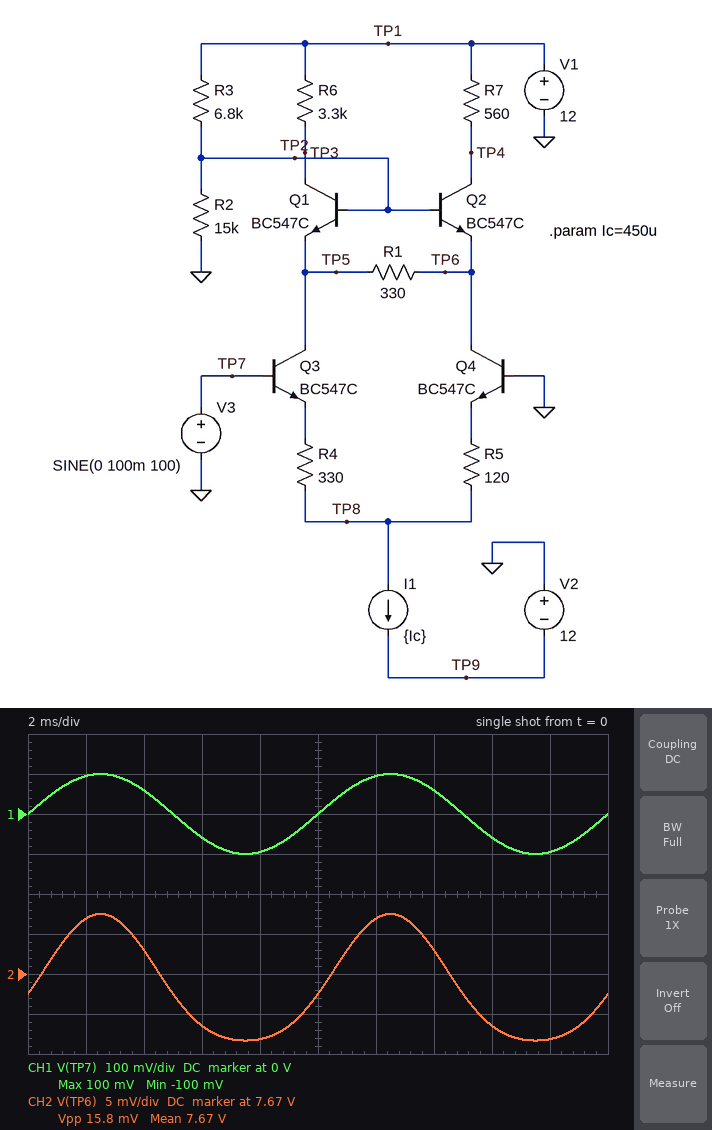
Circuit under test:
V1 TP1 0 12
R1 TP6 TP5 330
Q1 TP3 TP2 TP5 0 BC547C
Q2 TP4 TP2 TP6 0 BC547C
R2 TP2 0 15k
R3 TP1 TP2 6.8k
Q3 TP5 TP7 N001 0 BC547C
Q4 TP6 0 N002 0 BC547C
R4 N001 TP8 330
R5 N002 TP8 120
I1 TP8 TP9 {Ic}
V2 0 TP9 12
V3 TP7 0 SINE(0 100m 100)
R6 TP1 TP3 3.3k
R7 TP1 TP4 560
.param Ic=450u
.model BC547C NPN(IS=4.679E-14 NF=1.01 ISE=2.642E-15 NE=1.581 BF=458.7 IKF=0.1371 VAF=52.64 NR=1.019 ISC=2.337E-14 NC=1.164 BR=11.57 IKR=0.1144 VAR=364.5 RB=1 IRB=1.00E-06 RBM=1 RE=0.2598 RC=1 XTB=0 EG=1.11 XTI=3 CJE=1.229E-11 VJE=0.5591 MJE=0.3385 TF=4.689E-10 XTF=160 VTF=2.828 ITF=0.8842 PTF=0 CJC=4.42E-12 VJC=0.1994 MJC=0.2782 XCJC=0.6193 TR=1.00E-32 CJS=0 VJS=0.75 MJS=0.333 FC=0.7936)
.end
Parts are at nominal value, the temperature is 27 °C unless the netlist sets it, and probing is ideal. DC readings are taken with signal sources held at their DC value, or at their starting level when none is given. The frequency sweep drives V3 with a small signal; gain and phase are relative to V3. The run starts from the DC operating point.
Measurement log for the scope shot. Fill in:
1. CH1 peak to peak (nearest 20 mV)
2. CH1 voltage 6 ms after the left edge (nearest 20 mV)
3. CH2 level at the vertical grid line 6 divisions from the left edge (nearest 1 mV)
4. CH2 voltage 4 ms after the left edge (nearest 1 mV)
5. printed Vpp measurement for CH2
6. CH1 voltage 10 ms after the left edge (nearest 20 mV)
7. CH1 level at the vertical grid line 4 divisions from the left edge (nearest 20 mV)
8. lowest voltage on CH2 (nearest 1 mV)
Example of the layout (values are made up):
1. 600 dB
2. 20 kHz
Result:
1. 200 mV
2. -60 mV
3. 7.677 V
4. 7.673 V
5. 15.8 mV
6. 0 V
7. -100 mV
8. 7.662 V
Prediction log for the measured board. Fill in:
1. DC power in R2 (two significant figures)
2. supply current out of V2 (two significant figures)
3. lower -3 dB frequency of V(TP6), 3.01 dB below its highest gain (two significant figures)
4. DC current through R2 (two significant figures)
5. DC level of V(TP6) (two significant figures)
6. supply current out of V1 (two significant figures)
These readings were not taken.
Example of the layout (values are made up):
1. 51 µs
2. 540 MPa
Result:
1. 4.5 mW
2. 450 µA
3. 6.5 MHz
4. 550 µA
5. 7.7 V
6. 1.0 mA
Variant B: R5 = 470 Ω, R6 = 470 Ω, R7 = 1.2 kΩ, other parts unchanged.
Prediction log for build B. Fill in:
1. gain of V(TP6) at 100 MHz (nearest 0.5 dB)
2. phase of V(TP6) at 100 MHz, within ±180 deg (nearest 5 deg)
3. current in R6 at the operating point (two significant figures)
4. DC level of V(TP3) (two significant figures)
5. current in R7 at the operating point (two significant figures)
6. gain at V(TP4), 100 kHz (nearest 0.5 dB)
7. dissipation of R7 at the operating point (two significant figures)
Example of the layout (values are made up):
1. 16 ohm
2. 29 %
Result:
1. -11.0 dB
2. 35 deg
3. 240 µA
4. 12 V
5. 210 µA
6. -3.5 dB
7. 51 µW
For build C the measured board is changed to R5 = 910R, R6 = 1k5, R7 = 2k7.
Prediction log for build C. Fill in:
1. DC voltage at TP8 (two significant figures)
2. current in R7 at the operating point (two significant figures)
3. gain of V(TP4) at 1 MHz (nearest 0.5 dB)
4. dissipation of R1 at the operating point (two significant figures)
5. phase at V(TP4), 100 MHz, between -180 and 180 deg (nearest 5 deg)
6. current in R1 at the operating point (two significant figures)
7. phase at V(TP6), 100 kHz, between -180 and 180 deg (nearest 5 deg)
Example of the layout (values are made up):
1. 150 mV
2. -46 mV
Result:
1. -690 mV
2. 170 µA
3. 0 dB
4. 440 nW
5. 70 deg
6. 37 µA
7. 5 deg
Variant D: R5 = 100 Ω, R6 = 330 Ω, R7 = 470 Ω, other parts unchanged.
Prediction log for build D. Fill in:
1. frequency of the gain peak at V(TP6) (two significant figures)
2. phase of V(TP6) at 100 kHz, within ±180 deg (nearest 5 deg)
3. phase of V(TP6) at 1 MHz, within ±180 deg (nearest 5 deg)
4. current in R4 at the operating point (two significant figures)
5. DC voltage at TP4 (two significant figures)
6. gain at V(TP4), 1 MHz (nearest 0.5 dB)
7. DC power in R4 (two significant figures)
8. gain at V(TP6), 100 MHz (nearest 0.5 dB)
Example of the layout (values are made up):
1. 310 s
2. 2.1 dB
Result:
1. 25 MHz
2. 0 deg
3. -20 deg
4. 150 µA
5. 12 V
6. -8.0 dB
7. 7.2 µW
8. -13.5 dB
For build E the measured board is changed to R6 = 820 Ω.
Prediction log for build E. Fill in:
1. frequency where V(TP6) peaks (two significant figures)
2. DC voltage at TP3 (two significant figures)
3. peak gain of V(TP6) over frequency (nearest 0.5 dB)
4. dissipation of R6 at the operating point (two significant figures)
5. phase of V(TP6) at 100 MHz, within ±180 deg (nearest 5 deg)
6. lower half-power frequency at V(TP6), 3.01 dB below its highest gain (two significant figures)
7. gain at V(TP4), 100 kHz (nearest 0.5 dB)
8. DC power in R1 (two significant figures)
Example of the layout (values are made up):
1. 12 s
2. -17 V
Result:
1. 25 MHz
2. 12 V
3. -4.5 dB
4. 28 µW
5. -5 deg
6. 12 MHz
7. -7.0 dB
8. 270 nW
